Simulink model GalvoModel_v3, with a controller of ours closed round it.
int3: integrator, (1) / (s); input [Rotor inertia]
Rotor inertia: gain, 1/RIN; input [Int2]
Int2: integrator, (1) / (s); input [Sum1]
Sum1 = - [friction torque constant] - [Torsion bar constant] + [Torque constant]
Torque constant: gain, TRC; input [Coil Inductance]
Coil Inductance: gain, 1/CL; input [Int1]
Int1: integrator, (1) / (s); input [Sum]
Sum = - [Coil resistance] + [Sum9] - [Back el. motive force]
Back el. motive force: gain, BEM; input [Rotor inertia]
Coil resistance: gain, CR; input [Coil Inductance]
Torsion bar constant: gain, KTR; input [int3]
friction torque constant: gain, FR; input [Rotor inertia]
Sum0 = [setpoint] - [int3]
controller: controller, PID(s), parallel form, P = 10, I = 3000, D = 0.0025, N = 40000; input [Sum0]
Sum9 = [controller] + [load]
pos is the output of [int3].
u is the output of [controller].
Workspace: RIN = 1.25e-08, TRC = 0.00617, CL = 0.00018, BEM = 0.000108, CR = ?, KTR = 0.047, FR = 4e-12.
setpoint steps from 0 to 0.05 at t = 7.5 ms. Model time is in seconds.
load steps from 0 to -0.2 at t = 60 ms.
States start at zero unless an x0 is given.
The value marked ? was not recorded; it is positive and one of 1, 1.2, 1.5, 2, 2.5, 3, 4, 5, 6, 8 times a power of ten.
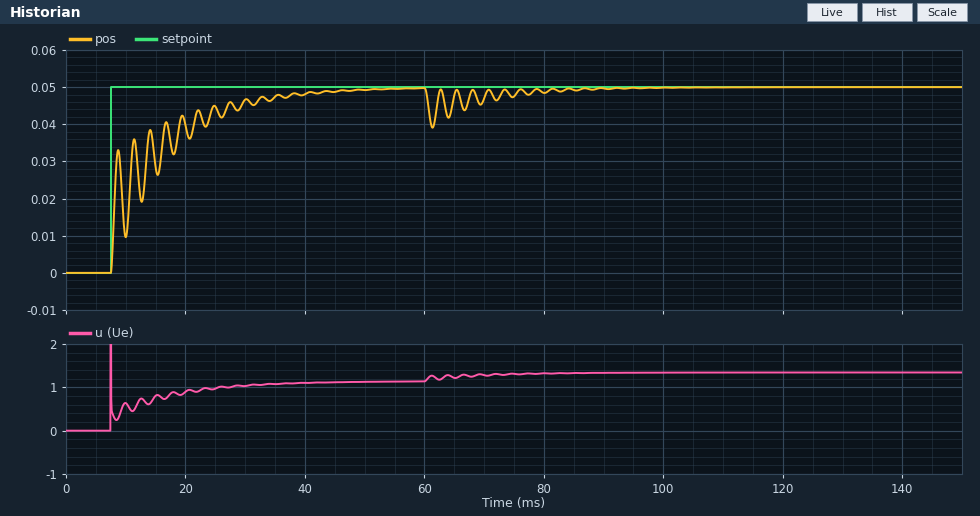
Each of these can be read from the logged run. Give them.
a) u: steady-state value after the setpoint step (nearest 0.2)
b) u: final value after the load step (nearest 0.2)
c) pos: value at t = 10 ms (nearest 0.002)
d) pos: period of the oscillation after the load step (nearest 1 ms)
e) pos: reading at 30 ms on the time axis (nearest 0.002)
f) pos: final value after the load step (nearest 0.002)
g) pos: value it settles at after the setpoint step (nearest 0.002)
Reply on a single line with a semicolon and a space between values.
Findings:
1.2; 1.4; 0.010; 3 ms; 0.046; 0.050; 0.050
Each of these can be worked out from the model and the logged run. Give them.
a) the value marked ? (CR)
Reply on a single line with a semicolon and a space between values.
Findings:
3
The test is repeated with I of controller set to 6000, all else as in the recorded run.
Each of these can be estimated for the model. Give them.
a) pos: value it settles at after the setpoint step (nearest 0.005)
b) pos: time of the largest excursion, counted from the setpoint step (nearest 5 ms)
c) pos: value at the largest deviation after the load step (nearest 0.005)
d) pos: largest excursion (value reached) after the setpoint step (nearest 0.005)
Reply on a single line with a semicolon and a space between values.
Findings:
0.050; 15 ms; 0.040; 0.055
